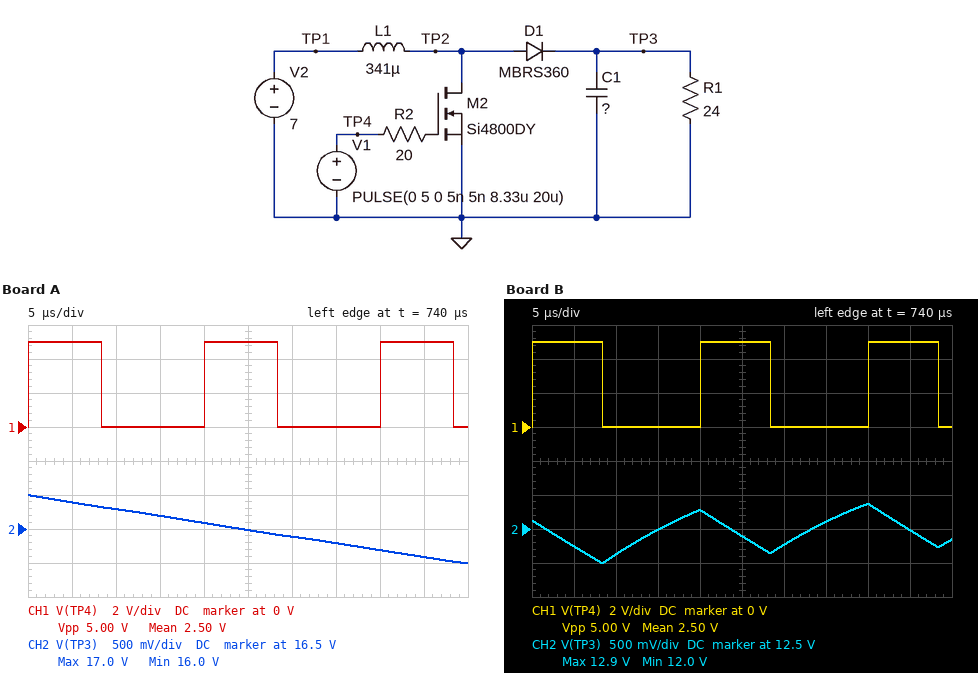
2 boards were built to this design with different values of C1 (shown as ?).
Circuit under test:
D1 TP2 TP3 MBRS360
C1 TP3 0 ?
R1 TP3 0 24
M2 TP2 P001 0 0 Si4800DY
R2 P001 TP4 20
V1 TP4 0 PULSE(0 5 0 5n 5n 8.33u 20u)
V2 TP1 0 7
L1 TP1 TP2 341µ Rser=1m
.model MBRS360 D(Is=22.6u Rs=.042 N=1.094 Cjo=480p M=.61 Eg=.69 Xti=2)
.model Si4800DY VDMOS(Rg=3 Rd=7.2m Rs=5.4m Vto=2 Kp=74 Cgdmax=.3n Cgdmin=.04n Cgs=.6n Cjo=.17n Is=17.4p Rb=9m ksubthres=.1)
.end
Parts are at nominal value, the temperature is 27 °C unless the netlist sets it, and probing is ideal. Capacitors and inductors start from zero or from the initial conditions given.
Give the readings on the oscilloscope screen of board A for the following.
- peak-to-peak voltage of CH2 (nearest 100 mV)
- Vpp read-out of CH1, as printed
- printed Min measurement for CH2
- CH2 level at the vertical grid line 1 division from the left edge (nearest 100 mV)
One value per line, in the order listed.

1.0 V
5.00 V
16.0 V
16.9 V
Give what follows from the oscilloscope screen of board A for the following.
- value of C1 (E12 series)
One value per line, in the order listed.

33 µF
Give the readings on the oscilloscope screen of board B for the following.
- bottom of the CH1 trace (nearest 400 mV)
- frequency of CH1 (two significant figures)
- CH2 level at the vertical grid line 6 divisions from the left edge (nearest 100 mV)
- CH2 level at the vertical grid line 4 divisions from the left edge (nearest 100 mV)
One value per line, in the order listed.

0 V
50 kHz
12.3 V
12.8 V
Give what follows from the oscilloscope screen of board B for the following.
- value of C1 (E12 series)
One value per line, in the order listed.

6.8 µF
